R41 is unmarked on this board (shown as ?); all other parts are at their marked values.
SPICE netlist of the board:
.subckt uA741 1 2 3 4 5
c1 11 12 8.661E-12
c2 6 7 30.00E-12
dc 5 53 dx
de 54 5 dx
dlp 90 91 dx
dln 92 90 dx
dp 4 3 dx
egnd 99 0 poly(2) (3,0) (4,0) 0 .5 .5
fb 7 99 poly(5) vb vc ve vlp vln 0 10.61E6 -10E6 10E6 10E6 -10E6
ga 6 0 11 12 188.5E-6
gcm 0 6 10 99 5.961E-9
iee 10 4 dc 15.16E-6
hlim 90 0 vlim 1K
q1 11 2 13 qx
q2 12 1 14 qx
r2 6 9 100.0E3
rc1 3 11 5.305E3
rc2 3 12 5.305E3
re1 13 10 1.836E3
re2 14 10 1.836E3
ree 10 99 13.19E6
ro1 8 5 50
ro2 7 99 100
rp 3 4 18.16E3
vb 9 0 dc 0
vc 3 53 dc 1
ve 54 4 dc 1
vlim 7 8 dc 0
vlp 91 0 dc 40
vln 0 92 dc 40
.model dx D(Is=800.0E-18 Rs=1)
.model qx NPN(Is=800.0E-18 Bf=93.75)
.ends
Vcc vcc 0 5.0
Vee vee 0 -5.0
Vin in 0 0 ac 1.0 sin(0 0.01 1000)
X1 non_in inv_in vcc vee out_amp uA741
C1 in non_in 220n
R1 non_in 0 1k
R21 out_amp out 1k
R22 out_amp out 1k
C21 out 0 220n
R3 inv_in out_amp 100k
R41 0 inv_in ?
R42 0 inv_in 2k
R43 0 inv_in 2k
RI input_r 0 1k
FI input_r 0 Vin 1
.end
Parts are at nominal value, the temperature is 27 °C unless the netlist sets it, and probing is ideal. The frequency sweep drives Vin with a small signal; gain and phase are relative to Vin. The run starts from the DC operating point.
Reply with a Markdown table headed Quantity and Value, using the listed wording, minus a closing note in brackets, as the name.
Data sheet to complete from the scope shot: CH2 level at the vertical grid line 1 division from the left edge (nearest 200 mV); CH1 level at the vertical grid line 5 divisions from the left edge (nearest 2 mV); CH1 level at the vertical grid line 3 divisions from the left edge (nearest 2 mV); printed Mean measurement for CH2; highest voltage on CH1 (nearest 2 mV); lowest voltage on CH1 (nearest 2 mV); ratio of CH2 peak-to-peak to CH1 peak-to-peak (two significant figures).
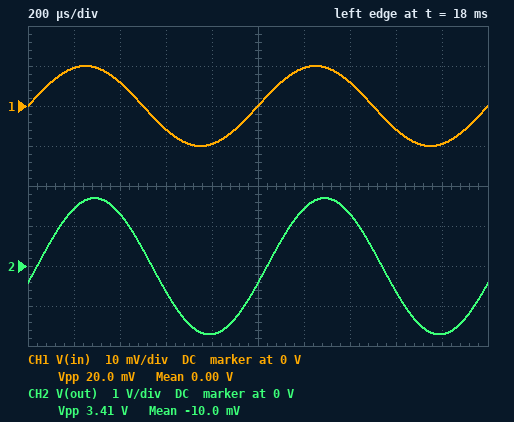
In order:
| Quantity | Value |
|---|---|
| CH2 level at the vertical grid line 1 division from the left edge | 1.4 V |
| CH1 level at the vertical grid line 5 divisions from the left edge | 0 V |
| CH1 level at the vertical grid line 3 divisions from the left edge | -6 mV |
| printed Mean measurement for CH2 | -10.0 mV |
| highest voltage on CH1 | 10 mV |
| lowest voltage on CH1 | -10 mV |
| ratio of CH2 peak-to-peak to CH1 peak-to-peak | 170 |
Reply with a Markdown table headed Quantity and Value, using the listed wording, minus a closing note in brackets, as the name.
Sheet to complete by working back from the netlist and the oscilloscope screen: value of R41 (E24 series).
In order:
| Quantity | Value |
|---|---|
| value of R41 | 620 Ω |
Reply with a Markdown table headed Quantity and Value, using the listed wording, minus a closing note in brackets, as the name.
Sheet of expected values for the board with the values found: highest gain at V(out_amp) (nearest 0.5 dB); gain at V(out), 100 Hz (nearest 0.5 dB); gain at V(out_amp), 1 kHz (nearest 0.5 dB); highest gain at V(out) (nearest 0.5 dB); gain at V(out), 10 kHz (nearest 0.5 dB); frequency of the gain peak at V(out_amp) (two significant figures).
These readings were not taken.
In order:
| Quantity | Value |
|---|---|
| highest gain at V(out_amp) | 47.0 dB |
| gain at V(out), 100 Hz | 31.0 dB |
| gain at V(out_amp), 1 kHz | 46.5 dB |
| highest gain at V(out) | 44.5 dB |
| gain at V(out), 10 kHz | 22.0 dB |
| frequency of the gain peak at V(out_amp) | 1.6 kHz |
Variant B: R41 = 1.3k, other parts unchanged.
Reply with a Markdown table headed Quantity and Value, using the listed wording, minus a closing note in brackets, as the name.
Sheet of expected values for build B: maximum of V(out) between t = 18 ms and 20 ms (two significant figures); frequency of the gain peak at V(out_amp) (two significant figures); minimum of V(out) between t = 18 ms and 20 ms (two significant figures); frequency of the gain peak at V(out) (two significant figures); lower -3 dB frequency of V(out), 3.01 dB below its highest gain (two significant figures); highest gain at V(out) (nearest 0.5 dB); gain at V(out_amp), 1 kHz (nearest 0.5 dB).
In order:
| Quantity | Value |
|---|---|
| maximum of V(out) between t = 18 ms and 20 ms | 1.2 V |
| frequency of the gain peak at V(out_amp) | 2.0 kHz |
| minimum of V(out) between t = 18 ms and 20 ms | -1.2 V |
| frequency of the gain peak at V(out) | 1.0 kHz |
| lower -3 dB frequency of V(out), 3.01 dB below its highest gain | 400 Hz |
| highest gain at V(out) | 41.5 dB |
| gain at V(out_amp), 1 kHz | 43.0 dB |
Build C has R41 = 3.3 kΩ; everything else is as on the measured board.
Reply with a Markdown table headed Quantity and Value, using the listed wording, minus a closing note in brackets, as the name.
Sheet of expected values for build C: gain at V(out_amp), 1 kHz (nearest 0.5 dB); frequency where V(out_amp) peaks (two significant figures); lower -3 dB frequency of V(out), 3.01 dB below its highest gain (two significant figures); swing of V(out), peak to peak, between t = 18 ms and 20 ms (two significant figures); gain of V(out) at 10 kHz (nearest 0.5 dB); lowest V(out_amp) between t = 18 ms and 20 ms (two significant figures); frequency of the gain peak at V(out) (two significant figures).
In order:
| Quantity | Value |
|---|---|
| gain at V(out_amp), 1 kHz | 40.5 dB |
| frequency where V(out_amp) peaks | 2.3 kHz |
| lower -3 dB frequency of V(out), 3.01 dB below its highest gain | 400 Hz |
| swing of V(out), peak to peak, between t = 18 ms and 20 ms | 1.7 V |
| gain of V(out) at 10 kHz | 20.5 dB |
| lowest V(out_amp) between t = 18 ms and 20 ms | -1.1 V |
| frequency of the gain peak at V(out) | 1.0 kHz |
